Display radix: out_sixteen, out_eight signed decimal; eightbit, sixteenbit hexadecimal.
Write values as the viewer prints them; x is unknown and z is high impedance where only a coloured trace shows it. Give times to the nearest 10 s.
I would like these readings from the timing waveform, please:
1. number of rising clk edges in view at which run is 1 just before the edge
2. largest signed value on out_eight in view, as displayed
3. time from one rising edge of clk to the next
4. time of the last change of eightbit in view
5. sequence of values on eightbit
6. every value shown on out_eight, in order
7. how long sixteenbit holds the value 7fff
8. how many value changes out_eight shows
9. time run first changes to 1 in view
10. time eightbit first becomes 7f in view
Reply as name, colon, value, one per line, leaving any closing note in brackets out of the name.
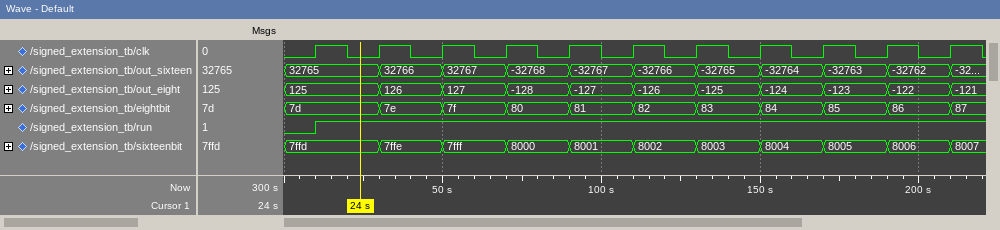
number of rising clk edges in view at which run is 1 just before the edge: 10
largest signed value on out_eight in view, as displayed: 127
time from one rising edge of clk to the next: 20 s
time of the last change of eightbit in view: 210 s
sequence of values on eightbit: 7d, 7e, 7f, 80, 81, 82, 83, 84, 85, 86, 87
every value shown on out_eight, in order: 125, 126, 127, -128, -127, -126, -125, -124, -123, -122, -121
how long sixteenbit holds the value 7fff: 20 s
how many value changes out_eight shows: 10
time run first changes to 1 in view: 10 s
time eightbit first becomes 7f in view: 50 s
